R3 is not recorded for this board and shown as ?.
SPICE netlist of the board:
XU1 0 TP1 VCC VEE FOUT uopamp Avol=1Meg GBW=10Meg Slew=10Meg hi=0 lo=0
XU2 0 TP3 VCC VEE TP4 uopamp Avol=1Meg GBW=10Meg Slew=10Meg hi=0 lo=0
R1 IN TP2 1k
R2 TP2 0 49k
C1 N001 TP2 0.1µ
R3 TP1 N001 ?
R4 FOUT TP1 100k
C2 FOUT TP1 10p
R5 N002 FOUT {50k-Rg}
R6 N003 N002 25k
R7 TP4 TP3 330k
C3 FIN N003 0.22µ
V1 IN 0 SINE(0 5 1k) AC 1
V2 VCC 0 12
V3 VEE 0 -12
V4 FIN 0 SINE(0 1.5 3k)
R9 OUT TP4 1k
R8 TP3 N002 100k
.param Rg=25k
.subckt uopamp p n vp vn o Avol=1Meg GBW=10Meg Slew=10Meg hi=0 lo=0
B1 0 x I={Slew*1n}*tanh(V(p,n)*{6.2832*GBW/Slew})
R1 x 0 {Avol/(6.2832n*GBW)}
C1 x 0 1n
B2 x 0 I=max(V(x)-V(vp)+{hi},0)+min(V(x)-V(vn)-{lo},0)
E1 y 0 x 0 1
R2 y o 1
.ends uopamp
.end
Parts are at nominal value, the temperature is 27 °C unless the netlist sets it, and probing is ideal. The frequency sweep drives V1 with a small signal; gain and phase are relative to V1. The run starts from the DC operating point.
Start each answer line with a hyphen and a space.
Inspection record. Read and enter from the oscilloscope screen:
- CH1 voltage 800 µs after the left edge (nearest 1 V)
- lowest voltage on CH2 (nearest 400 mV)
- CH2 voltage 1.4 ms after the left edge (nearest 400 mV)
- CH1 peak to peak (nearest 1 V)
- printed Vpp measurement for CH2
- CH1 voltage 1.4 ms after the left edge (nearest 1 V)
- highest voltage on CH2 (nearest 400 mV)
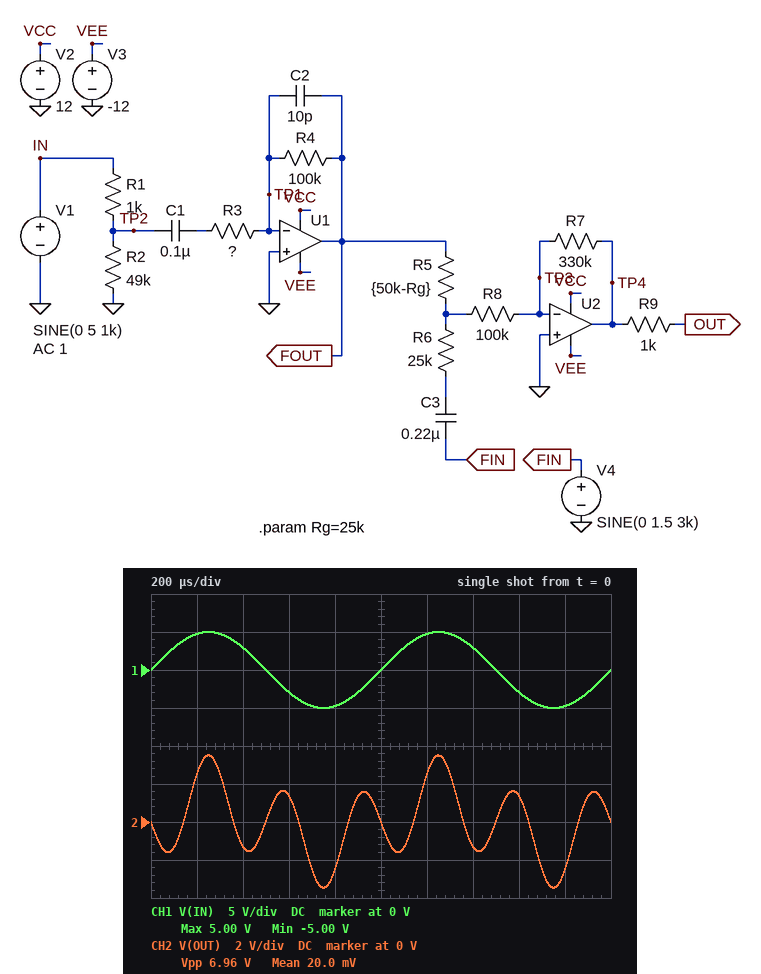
- -5 V
- -3.6 V
- -1.2 V
- 10 V
- 6.96 V
- 3 V
- 3.6 V
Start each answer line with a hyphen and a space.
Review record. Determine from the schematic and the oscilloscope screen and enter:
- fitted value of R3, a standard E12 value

- 560 kΩ
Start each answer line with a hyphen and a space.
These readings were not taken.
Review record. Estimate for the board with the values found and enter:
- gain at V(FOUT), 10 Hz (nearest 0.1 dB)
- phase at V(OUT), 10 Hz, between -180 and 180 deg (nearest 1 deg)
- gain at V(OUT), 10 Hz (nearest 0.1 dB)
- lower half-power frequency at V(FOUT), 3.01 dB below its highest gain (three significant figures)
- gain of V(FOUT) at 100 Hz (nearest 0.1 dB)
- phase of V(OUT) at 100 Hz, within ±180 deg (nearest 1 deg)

- -15.5 dB
- 3 deg
- -8.0 dB
- 2.84 Hz
- -15.2 dB
- -5 deg
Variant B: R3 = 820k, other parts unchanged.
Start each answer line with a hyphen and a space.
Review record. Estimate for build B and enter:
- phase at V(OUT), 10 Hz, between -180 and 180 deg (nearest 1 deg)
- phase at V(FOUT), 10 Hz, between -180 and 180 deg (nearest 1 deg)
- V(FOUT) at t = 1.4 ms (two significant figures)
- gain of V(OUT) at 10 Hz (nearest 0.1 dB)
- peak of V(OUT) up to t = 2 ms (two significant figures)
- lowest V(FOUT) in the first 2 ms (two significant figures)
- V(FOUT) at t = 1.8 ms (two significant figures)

- -2 deg
- -169 deg
- -350 mV
- -11.1 dB
- 3.1 V
- -600 mV
- 570 mV
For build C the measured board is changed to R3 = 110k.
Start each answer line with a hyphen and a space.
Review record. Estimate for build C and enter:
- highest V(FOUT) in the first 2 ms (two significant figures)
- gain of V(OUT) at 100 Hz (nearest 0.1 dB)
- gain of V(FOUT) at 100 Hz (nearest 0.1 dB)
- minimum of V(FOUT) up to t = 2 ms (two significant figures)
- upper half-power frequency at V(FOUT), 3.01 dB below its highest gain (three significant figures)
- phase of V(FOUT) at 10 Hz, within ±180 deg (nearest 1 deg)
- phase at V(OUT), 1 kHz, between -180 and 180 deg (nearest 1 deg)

- 4.5 V
- 2.4 dB
- -1.2 dB
- -4.4 V
- 157 kHz
- -125 deg
- 0 deg
